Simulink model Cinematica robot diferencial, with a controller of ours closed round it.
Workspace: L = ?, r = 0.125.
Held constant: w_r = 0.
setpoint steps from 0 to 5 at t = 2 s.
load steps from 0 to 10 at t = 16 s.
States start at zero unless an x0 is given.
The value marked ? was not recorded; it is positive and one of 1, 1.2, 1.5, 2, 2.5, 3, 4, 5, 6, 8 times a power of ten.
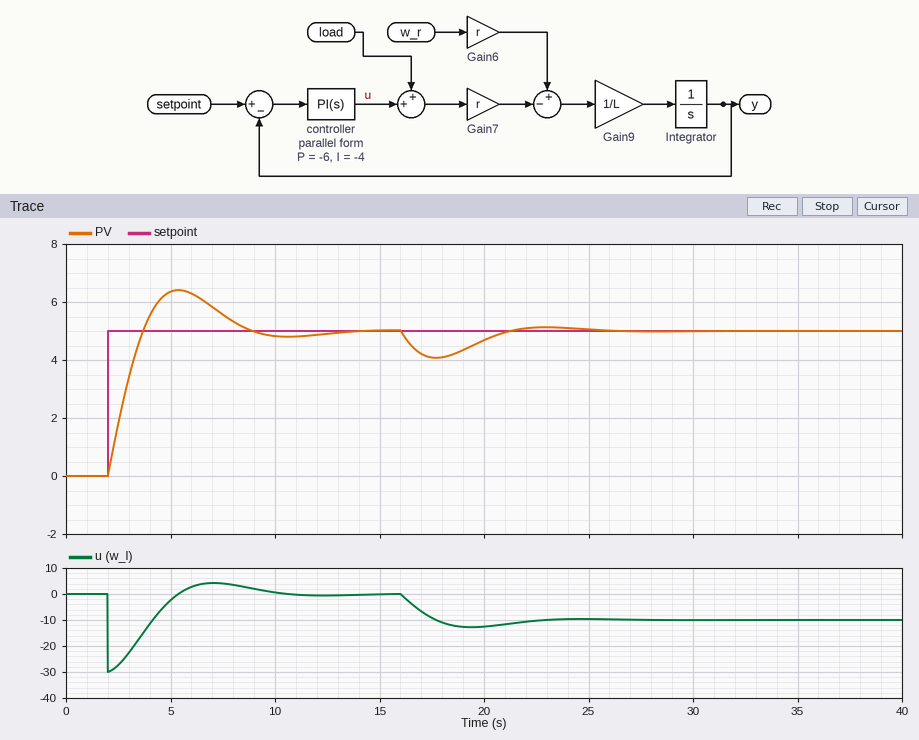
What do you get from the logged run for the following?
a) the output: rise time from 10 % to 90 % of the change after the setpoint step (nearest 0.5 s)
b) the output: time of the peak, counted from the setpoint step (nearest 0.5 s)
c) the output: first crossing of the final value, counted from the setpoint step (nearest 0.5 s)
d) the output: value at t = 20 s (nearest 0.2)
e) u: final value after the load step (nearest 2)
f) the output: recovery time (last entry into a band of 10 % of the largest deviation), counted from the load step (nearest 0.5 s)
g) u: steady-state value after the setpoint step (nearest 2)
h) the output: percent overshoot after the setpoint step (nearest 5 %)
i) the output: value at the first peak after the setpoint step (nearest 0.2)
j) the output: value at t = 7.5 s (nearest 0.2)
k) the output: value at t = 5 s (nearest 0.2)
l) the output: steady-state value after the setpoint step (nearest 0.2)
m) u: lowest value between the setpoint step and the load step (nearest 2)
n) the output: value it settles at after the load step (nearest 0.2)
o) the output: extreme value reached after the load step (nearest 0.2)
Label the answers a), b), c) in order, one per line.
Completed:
a) 1.5 s
b) 3.5 s
c) 1.5 s
d) 4.6
e) -10
f) 8.0 s
g) 0
h) 30 %
i) 6.4
j) 5.6
k) 6.4
l) 5.0
m) -30
n) 5.0
o) 4.0
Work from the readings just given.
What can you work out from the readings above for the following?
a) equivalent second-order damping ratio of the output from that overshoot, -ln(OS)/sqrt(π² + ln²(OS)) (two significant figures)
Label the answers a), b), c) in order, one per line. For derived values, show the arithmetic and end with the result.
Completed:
a) ln(0.3) = -1.204; 1.204 / sqrt(9.870 + 1.450) = 0.36
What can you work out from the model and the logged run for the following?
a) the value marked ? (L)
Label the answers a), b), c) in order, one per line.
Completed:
a) 1
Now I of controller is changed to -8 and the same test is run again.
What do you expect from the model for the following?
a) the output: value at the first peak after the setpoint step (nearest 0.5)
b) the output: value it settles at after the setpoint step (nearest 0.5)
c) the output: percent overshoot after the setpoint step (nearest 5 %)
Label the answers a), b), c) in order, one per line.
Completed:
a) 7.0
b) 5.0
c) 40 %
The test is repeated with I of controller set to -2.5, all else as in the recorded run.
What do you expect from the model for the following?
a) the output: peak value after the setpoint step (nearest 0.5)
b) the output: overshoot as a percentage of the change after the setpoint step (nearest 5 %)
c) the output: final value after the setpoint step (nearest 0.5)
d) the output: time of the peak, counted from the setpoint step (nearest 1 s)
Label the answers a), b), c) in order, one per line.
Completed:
a) 6.0
b) 20 %
c) 5.0
d) 4 s
